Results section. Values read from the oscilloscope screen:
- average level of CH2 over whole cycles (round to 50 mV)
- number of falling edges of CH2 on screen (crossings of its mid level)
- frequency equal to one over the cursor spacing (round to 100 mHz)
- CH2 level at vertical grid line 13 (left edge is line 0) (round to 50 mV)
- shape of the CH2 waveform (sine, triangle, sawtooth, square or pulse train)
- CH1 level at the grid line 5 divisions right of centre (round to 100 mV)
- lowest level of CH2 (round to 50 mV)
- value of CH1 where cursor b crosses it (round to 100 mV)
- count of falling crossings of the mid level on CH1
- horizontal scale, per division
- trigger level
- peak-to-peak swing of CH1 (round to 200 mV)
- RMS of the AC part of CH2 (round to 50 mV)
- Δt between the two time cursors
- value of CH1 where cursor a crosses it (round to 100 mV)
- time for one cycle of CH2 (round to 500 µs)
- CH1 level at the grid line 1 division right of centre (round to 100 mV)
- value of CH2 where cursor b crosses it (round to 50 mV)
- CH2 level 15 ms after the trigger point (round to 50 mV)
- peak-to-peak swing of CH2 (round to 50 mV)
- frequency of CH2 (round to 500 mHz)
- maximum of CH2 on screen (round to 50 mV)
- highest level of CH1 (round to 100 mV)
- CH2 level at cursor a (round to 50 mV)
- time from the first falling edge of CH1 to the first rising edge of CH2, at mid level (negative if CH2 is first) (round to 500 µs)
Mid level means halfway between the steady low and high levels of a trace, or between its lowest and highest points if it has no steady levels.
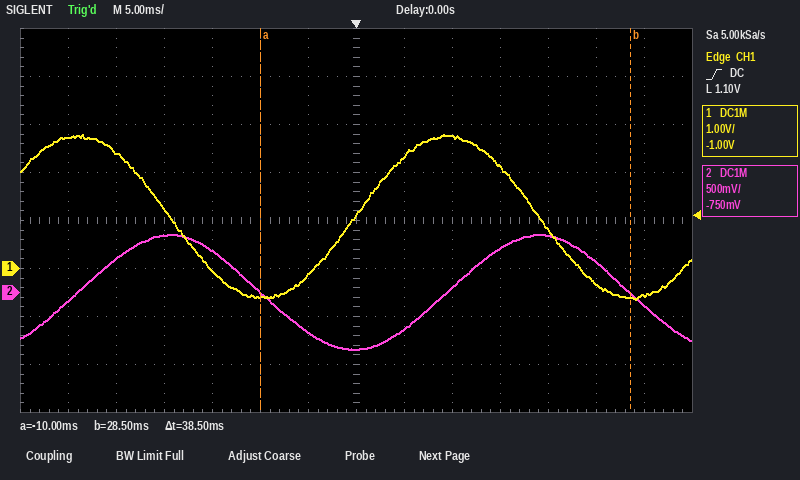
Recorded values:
0 mV
2
26.0 Hz
-150 mV
sine
-300 mV
-600 mV
-600 mV
2
5 ms
1.10 V
3.4 V
400 mV
38.5 ms
-600 mV
38.5 ms
2.3 V
0 mV
450 mV
1.20 V
26.0 Hz
600 mV
2.8 V
0 mV
-9.5 ms
